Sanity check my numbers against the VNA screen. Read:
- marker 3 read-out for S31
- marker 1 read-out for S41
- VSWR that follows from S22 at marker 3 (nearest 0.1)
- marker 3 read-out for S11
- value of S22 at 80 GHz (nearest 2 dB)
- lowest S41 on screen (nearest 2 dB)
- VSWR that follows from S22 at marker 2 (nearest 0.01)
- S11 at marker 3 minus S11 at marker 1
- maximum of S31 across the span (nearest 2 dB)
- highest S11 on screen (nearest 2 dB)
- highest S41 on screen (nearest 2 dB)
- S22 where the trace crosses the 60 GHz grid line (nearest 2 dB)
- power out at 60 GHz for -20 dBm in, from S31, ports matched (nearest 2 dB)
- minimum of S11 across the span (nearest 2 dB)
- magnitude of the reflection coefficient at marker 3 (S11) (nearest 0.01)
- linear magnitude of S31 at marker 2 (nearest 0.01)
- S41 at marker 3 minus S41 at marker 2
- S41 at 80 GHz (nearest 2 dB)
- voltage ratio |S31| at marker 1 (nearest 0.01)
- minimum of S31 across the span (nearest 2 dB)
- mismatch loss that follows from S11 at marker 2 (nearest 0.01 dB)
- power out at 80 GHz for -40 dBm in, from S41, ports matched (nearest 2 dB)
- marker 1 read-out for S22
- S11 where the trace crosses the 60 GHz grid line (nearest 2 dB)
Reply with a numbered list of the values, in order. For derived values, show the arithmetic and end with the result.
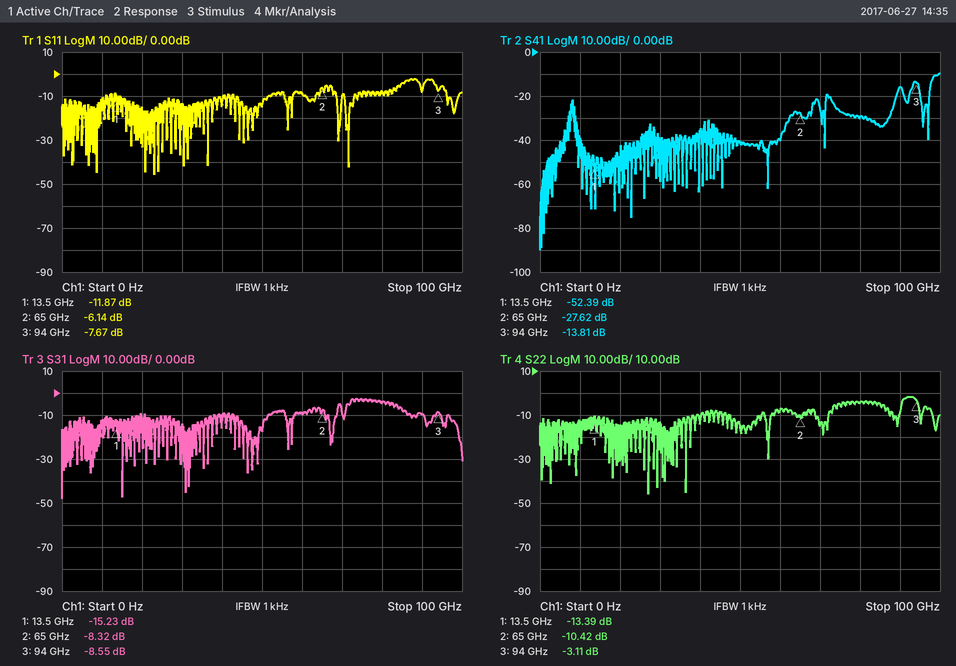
1. -8.55 dB
2. -52.39 dB
3. (1 + 0.6990)/(1 − 0.6990) ≈ 5.6
4. -7.67 dB
5. -4 dB
6. -90 dB
7. (1 + 0.3013)/(1 − 0.3013) ≈ 1.86
8. -7.67 − (-11.87) = 4.20 dB
9. -2 dB
10. -2 dB
11. -10 dB
12. -8 dB
13. -20 dBm + (-10 dB) = -30 dBm
14. -46 dB
15. 10^(-7.67/20) ≈ 0.41
16. 10^(-8.32/20) ≈ 0.38
17. -13.81 − (-27.62) = 13.81 dB
18. -30 dB
19. 10^(-15.23/20) ≈ 0.17
20. -48 dB
21. −10 log10(1 − 10^(-6.14/10)) ≈ 1.21 dB
22. -40 dBm + (-30 dB) = -70 dBm
23. -13.39 dB
24. -8 dB
